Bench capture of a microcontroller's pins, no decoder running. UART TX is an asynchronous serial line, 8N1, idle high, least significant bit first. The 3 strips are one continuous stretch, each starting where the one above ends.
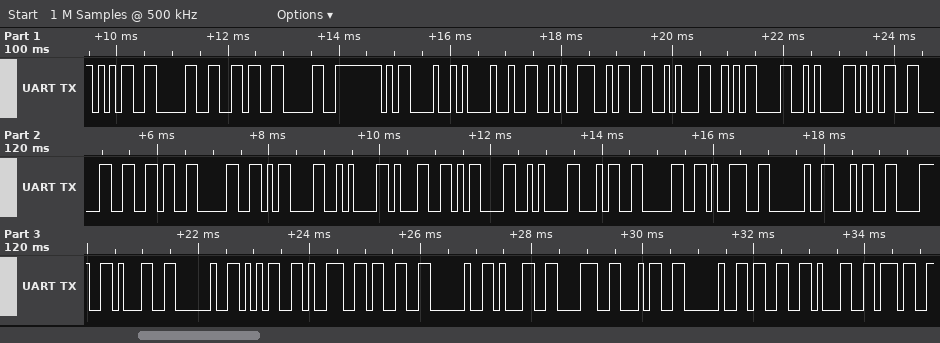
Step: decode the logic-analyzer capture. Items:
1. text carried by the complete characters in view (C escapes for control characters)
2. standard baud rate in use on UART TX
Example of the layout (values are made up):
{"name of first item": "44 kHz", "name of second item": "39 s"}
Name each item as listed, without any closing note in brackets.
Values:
{"text carried by the complete characters in view": "\"5060\\r\\n2931\\r\\n5060\\r\\n1\\r\\n409 481 593 184 317\"", "standard baud rate in use on UART TX": "9600 baud"}
